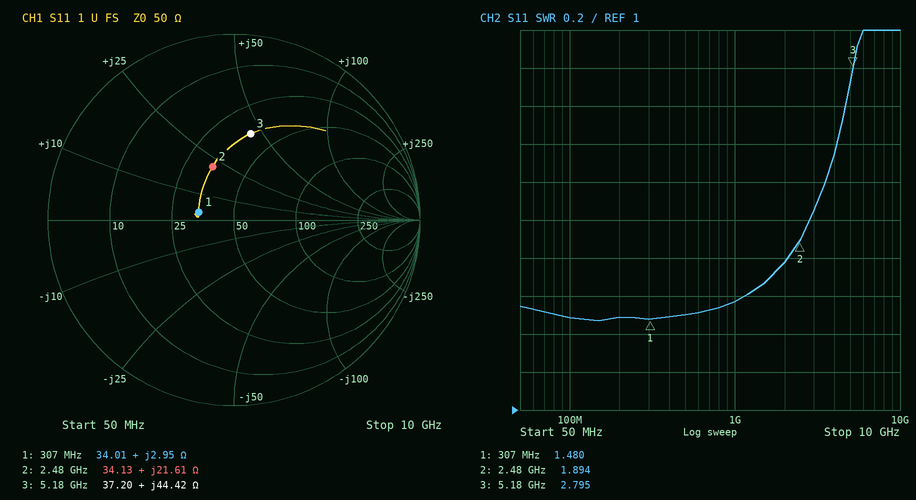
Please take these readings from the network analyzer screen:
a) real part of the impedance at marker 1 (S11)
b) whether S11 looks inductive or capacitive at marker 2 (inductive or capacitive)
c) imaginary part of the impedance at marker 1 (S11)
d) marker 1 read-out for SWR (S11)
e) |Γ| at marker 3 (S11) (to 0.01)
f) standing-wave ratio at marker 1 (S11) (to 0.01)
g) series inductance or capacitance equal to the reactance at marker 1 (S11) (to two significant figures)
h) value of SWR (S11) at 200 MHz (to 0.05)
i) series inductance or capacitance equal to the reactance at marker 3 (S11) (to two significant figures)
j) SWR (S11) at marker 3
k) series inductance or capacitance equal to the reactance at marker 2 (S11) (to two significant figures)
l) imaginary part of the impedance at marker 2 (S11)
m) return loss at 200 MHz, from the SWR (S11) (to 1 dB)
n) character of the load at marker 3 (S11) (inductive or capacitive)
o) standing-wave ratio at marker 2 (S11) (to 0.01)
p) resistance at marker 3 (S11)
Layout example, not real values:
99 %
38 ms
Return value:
34.01 Ω
inductive
+2.95 Ω
1.480
0.47
1.48
1.5 nH
1.50
1.4 nH
2.795
1.4 nH
+21.61 Ω
14 dB
inductive
1.89
37.20 Ω
